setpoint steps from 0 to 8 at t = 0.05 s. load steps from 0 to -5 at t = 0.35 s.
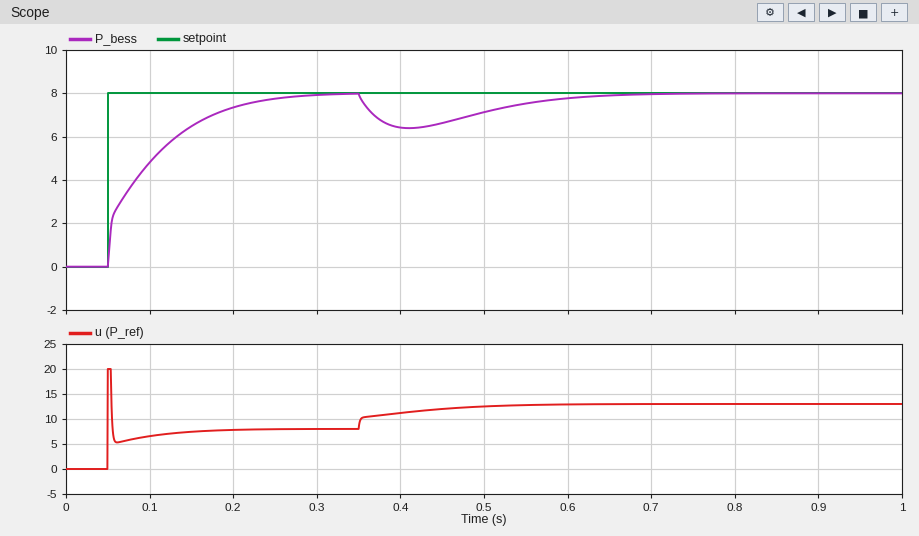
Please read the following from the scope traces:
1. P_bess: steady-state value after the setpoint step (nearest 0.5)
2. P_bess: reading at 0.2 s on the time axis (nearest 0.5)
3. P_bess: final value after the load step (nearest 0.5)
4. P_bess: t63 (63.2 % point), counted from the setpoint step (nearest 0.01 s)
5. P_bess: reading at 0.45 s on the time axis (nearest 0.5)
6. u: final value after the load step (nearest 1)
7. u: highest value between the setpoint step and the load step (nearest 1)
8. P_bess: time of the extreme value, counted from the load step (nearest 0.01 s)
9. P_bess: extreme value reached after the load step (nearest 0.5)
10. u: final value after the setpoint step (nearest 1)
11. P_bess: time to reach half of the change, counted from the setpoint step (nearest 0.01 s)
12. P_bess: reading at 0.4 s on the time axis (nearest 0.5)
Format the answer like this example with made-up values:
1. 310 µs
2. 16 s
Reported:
1. 8.0
2. 7.5
3. 8.0
4. 0.06 s
5. 6.5
6. 13
7. 20
8. 0.06 s
9. 6.5
10. 8
11. 0.03 s
12. 6.5
